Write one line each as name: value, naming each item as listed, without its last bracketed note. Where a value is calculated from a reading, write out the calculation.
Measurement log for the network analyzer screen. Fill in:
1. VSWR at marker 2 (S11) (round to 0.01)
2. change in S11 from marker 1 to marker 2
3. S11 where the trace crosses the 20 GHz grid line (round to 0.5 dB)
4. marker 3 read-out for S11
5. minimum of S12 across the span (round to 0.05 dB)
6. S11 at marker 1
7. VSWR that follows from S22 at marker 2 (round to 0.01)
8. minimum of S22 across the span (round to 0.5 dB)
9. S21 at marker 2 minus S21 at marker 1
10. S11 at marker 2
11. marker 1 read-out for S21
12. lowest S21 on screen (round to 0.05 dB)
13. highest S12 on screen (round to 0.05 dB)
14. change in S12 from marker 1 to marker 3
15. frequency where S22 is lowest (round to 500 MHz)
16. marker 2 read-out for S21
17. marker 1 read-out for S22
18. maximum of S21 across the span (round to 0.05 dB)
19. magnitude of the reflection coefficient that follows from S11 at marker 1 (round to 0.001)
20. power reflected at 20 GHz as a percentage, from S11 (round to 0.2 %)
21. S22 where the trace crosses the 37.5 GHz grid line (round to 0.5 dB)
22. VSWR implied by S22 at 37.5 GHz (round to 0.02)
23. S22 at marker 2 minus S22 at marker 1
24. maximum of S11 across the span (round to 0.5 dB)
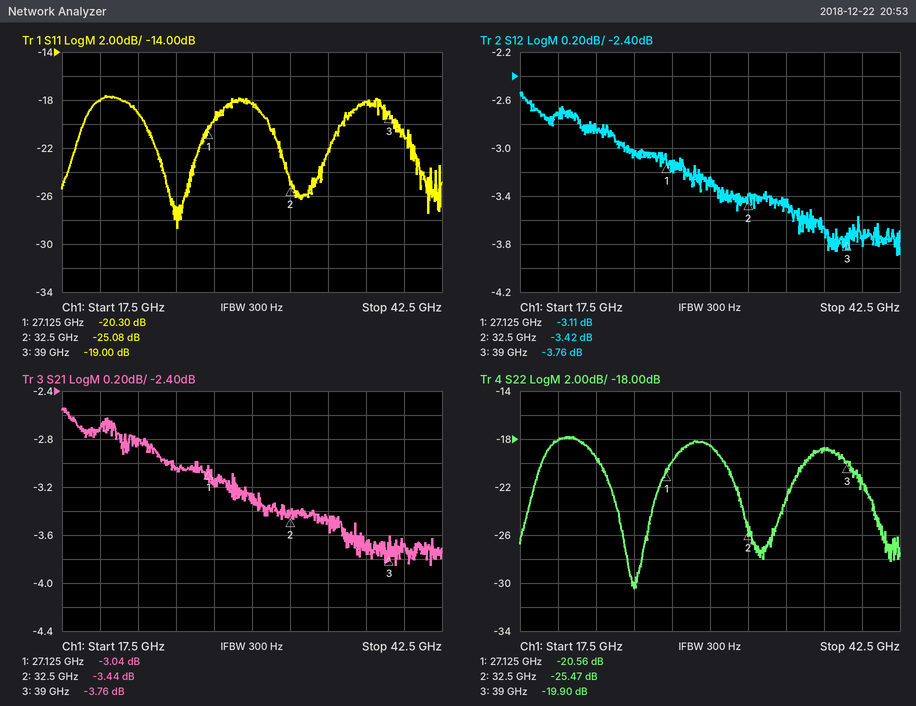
VSWR at marker 2 (S11): (1 + 0.0557)/(1 − 0.0557) ≈ 1.12
change in S11 from marker 1 to marker 2: -25.08 − (-20.3) = -4.78 dB
S11 where the trace crosses the 20 GHz grid line: -18.0 dB
marker 3 read-out for S11: -19.00 dB
minimum of S12 across the span: -3.90 dB
S11 at marker 1: -20.30 dB
VSWR that follows from S22 at marker 2: (1 + 0.0533)/(1 − 0.0533) ≈ 1.11
minimum of S22 across the span: -30.5 dB
S21 at marker 2 minus S21 at marker 1: -3.44 − (-3.04) = -0.40 dB
S11 at marker 2: -25.08 dB
marker 1 read-out for S21: -3.04 dB
lowest S21 on screen: -3.85 dB
highest S12 on screen: -2.55 dB
change in S12 from marker 1 to marker 3: -3.76 − (-3.11) = -0.65 dB
frequency where S22 is lowest: 25.0 GHz
marker 2 read-out for S21: -3.44 dB
marker 1 read-out for S22: -20.56 dB
maximum of S21 across the span: -2.55 dB
magnitude of the reflection coefficient that follows from S11 at marker 1: 10^(-20.3/20) ≈ 0.097
power reflected at 20 GHz as a percentage, from S11: 10^(-18/10) ≈ 1.6 %
S22 where the trace crosses the 37.5 GHz grid line: -19.0 dB
VSWR implied by S22 at 37.5 GHz: |Γ| = 10^(-19/20) = 0.1122; VSWR = (1 + 0.1122)/(1 − 0.1122) ≈ 1.25, so 1.26 to the nearest 0.02
S22 at marker 2 minus S22 at marker 1: -25.47 − (-20.56) = -4.91 dB
maximum of S11 across the span: -17.5 dB
